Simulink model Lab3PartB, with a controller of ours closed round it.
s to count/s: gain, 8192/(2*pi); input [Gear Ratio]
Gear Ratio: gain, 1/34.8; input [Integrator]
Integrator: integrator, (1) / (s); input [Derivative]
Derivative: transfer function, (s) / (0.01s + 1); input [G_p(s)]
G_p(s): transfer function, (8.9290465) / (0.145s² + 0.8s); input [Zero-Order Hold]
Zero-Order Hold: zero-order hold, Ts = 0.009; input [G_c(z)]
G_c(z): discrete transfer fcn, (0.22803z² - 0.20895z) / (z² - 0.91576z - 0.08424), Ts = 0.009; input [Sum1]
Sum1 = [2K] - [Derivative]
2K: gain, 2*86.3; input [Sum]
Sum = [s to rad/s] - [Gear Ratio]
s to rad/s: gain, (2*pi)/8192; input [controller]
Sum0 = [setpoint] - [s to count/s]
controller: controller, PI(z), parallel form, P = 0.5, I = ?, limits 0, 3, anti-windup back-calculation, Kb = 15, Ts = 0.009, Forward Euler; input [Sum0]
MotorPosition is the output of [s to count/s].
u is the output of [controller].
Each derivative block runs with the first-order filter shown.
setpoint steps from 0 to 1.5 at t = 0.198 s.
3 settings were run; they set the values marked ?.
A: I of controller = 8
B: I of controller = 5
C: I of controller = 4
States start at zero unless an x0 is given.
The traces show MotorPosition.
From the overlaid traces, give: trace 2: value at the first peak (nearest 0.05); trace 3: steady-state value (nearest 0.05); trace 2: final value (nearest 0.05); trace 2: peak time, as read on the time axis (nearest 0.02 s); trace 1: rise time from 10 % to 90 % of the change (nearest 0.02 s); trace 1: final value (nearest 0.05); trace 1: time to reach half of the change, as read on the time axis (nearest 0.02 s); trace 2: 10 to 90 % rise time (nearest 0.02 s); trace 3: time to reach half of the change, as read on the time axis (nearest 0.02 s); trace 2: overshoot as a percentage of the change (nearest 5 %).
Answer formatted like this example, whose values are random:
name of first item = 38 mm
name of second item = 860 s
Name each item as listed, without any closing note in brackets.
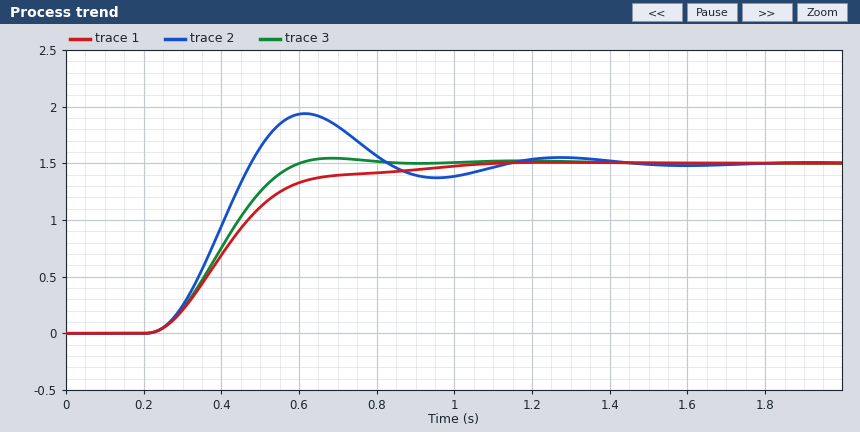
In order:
trace 2: value at the first peak = 1.95
trace 3: steady-state value = 1.50
trace 2: final value = 1.50
trace 2: peak time, as read on the time axis = 0.62 s
trace 1: rise time from 10 % to 90 % of the change = 0.34 s
trace 1: final value = 1.50
trace 1: time to reach half of the change, as read on the time axis = 0.42 s
trace 2: 10 to 90 % rise time = 0.18 s
trace 3: time to reach half of the change, as read on the time axis = 0.40 s
trace 2: overshoot as a percentage of the change = 30 %
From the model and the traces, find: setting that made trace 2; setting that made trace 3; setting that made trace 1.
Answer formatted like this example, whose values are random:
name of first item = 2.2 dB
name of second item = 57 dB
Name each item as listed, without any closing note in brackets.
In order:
setting that made trace 2 = A
setting that made trace 3 = B
setting that made trace 1 = C
